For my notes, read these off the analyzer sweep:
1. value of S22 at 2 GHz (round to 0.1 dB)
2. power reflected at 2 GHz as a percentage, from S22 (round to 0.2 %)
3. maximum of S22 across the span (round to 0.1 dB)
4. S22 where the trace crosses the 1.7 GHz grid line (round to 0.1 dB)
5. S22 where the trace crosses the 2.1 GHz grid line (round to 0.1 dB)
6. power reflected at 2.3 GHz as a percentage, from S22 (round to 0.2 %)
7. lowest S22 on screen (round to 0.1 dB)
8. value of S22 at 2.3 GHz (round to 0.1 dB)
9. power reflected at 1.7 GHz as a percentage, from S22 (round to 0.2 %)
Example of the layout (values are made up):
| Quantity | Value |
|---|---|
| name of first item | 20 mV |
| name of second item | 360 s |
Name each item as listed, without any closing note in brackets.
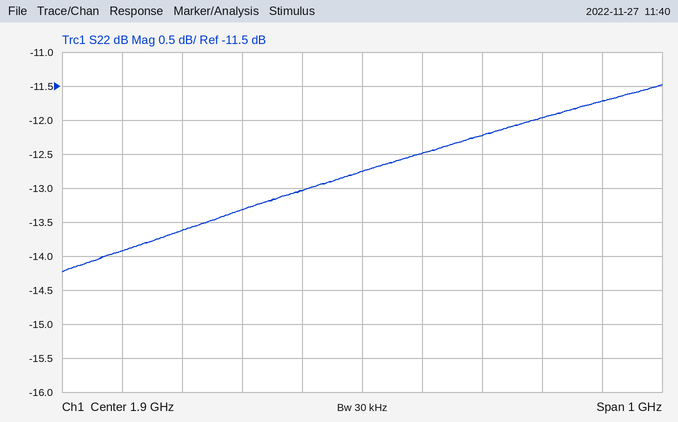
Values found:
| Quantity | Value |
|---|---|
| value of S22 at 2 GHz | -12.5 dB |
| power reflected at 2 GHz as a percentage, from S22 | 5.6 % |
| maximum of S22 across the span | -11.5 dB |
| S22 where the trace crosses the 1.7 GHz grid line | -13.3 dB |
| S22 where the trace crosses the 2.1 GHz grid line | -12.2 dB |
| power reflected at 2.3 GHz as a percentage, from S22 | 6.8 % |
| lowest S22 on screen | -14.2 dB |
| value of S22 at 2.3 GHz | -11.7 dB |
| power reflected at 1.7 GHz as a percentage, from S22 | 4.6 % |
